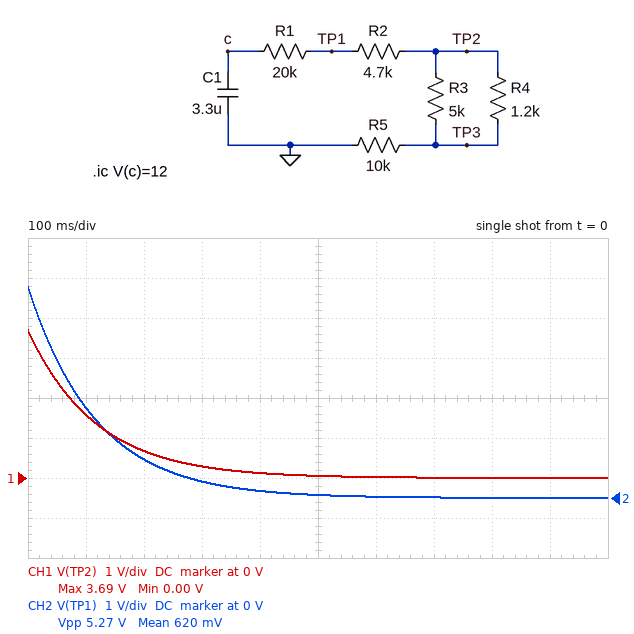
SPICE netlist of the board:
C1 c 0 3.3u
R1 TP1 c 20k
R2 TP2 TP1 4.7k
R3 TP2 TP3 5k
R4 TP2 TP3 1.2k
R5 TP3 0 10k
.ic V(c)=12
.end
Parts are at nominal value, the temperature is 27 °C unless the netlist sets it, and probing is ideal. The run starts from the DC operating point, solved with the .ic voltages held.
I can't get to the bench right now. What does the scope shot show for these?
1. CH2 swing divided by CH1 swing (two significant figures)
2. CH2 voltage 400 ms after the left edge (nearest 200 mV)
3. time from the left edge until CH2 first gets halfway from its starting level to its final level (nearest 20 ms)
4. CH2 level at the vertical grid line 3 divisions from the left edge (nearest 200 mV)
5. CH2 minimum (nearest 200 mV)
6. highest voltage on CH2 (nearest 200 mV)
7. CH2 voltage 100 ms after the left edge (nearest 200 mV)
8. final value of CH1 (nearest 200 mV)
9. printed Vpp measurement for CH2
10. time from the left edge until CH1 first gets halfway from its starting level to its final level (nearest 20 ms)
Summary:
1.4
200 mV
80 ms
400 mV
0 V
5.2 V
2.2 V
0 V
5.27 V
80 ms
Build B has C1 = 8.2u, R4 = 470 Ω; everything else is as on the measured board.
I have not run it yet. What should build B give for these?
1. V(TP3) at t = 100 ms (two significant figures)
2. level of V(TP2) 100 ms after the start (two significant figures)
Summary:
2.4 V
2.5 V
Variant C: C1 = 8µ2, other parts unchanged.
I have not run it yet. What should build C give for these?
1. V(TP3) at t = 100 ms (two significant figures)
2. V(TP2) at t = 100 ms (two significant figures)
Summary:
2.4 V
2.6 V
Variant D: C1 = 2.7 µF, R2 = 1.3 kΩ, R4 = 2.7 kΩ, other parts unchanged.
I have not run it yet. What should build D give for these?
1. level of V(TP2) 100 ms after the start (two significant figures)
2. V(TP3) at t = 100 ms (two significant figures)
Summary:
1.4 V
1.2 V
